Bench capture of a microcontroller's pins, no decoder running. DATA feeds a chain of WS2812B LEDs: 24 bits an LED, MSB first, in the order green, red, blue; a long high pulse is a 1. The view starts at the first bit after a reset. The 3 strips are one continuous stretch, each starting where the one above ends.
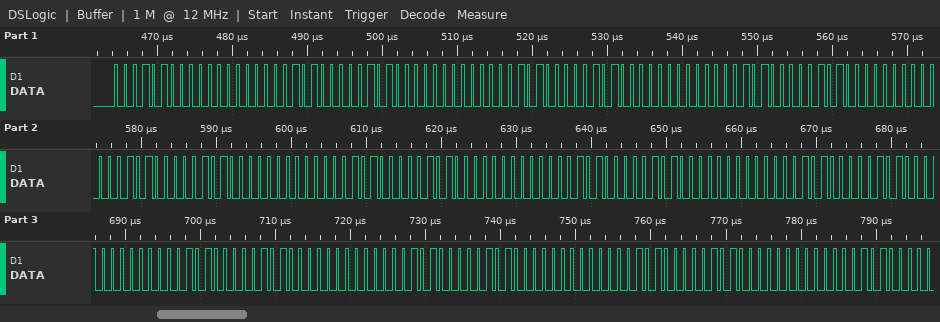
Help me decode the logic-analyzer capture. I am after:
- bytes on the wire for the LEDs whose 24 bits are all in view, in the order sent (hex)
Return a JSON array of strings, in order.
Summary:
["14 00 14 14 00 14 14 00 14 14 00 14 14 00 14 14 00 14 14 00 14 14 00 14 14 00 14 14 00 14 14 00 14"]
